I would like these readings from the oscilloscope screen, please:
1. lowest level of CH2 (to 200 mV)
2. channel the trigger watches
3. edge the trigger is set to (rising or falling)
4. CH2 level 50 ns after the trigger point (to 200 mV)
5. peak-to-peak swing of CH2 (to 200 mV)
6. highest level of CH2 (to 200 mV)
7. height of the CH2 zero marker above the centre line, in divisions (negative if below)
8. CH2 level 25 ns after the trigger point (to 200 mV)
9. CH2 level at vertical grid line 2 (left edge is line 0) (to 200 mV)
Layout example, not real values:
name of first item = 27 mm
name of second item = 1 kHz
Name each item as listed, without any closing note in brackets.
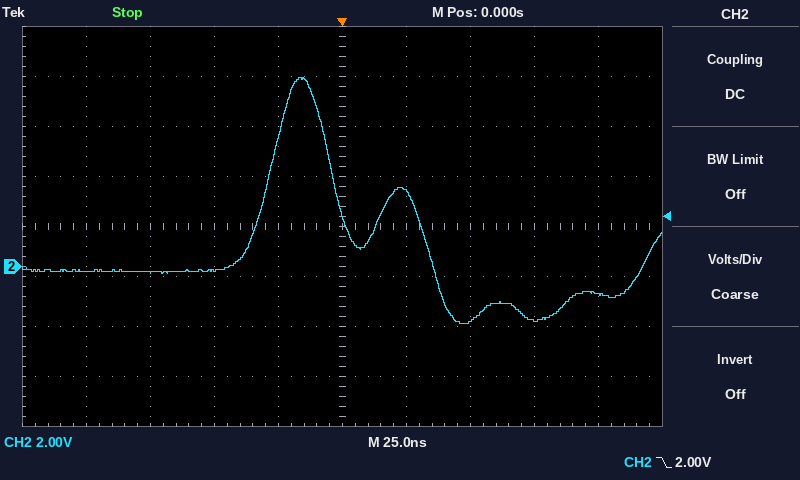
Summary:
lowest level of CH2 = -2.2 V
channel the trigger watches = CH2
edge the trigger is set to = falling
CH2 level 50 ns after the trigger point = -2.2 V
peak-to-peak swing of CH2 = 9.8 V
highest level of CH2 = 7.6 V
height of the CH2 zero marker above the centre line, in divisions = -0.8 div
CH2 level 25 ns after the trigger point = 3.0 V
CH2 level at vertical grid line 2 (left edge is line 0) = -200 mV
